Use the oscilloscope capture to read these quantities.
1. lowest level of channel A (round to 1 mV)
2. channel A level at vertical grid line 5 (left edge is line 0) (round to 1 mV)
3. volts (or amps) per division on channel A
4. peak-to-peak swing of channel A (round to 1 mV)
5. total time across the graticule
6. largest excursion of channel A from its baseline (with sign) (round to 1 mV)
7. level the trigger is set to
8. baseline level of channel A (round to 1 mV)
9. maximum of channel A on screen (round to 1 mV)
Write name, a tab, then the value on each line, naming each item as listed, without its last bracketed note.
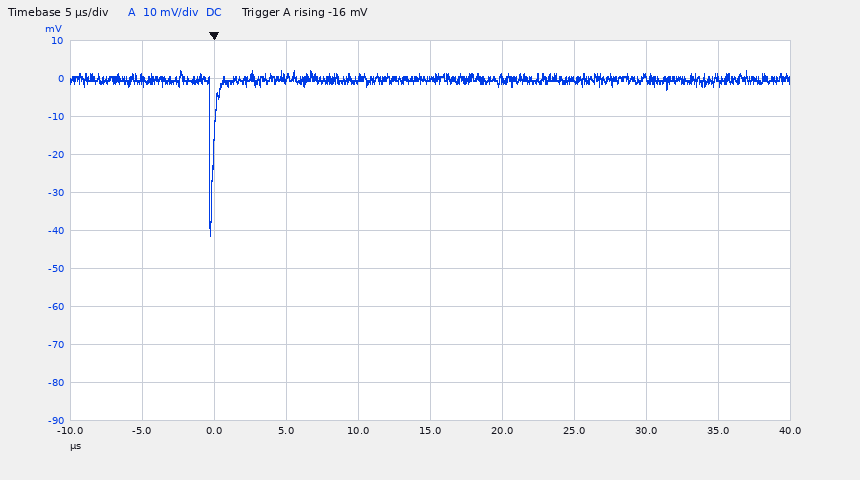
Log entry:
lowest level of channel A	-41 mV
channel A level at vertical grid line 5 (left edge is line 0)	0 mV
volts (or amps) per division on channel A	10 mV
peak-to-peak swing of channel A	43 mV
total time across the graticule	50 µs
largest excursion of channel A from its baseline (with sign)	-41 mV
level the trigger is set to	-16 mV
baseline level of channel A	0 mV
maximum of channel A on screen	2 mV
